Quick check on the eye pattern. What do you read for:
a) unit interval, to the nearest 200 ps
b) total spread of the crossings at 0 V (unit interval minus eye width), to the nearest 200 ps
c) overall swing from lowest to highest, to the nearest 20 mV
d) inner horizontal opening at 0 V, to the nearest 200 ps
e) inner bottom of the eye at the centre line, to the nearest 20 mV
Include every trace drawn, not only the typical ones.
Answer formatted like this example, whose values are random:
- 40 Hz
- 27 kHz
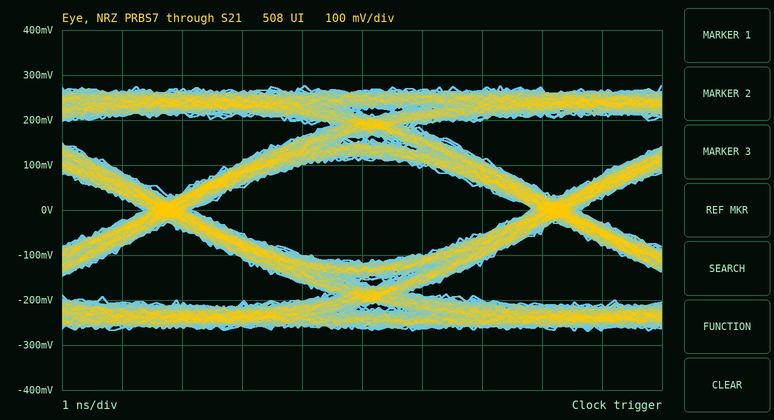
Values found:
- 6.4 ns
- 800 ps
- 540 mV
- 5.6 ns
- -120 mV
